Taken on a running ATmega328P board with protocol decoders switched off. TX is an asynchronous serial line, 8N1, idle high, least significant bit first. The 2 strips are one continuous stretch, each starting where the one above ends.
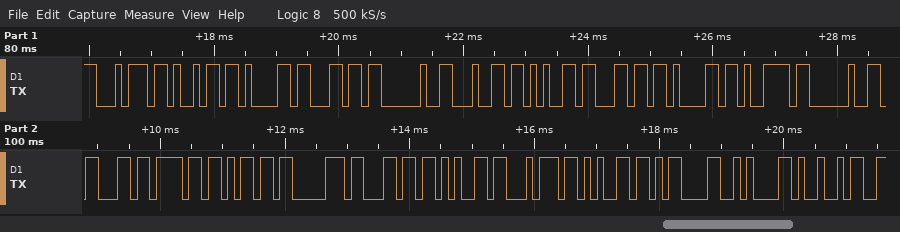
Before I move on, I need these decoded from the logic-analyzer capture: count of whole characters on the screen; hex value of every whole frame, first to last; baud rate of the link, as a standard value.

22
0x74 0x69 0x61 0x6C 0x20 0x64 0x65 0x6C 0x61 0x79 0x20 0x63 0x6F 0x6D 0x70 0x6C 0x65 0x74 0x65 0x0D 0x0A 0x49
9600 baud
